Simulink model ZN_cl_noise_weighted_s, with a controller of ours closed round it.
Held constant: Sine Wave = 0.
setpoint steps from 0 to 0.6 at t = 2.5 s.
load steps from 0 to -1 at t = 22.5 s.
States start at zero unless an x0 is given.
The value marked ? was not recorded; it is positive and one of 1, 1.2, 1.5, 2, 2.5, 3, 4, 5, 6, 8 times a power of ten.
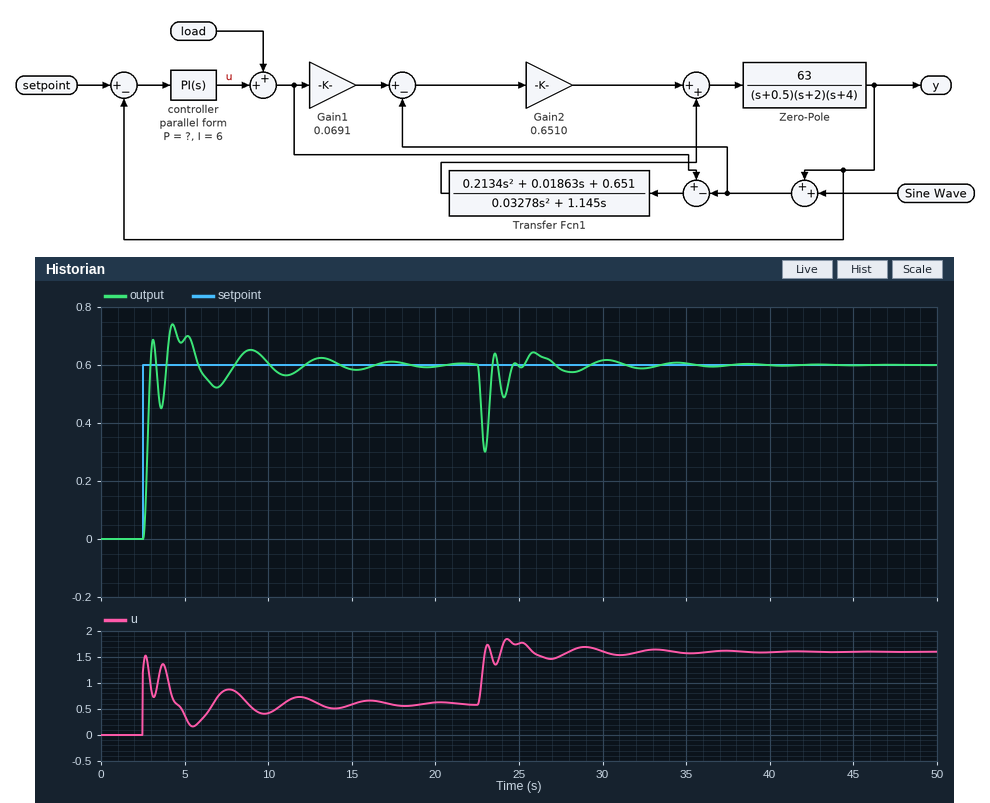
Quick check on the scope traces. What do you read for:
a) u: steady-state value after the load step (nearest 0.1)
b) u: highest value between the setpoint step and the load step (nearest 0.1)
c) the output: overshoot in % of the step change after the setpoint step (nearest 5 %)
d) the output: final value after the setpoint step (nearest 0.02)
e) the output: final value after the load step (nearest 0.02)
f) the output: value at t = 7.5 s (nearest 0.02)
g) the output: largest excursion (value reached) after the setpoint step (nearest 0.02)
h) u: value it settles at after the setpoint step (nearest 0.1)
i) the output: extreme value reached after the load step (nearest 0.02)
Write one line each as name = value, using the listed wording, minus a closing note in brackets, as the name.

u: steady-state value after the load step = 1.6
u: highest value between the setpoint step and the load step = 1.5
the output: overshoot in % of the step change after the setpoint step = 25 %
the output: final value after the setpoint step = 0.60
the output: final value after the load step = 0.60
the output: value at t = 7.5 s = 0.56
the output: largest excursion (value reached) after the setpoint step = 0.74
u: value it settles at after the setpoint step = 0.6
the output: extreme value reached after the load step = 0.30
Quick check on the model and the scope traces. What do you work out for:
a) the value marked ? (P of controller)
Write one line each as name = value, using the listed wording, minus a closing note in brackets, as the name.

the value marked ? = 2
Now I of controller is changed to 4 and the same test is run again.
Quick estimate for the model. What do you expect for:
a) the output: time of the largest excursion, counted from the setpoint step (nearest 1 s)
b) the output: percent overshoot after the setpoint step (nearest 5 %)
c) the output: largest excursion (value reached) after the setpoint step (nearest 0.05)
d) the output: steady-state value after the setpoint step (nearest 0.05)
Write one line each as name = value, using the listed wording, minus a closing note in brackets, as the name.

the output: time of the largest excursion, counted from the setpoint step = 3 s
the output: percent overshoot after the setpoint step = 20 %
the output: largest excursion (value reached) after the setpoint step = 0.70
the output: steady-state value after the setpoint step = 0.60
